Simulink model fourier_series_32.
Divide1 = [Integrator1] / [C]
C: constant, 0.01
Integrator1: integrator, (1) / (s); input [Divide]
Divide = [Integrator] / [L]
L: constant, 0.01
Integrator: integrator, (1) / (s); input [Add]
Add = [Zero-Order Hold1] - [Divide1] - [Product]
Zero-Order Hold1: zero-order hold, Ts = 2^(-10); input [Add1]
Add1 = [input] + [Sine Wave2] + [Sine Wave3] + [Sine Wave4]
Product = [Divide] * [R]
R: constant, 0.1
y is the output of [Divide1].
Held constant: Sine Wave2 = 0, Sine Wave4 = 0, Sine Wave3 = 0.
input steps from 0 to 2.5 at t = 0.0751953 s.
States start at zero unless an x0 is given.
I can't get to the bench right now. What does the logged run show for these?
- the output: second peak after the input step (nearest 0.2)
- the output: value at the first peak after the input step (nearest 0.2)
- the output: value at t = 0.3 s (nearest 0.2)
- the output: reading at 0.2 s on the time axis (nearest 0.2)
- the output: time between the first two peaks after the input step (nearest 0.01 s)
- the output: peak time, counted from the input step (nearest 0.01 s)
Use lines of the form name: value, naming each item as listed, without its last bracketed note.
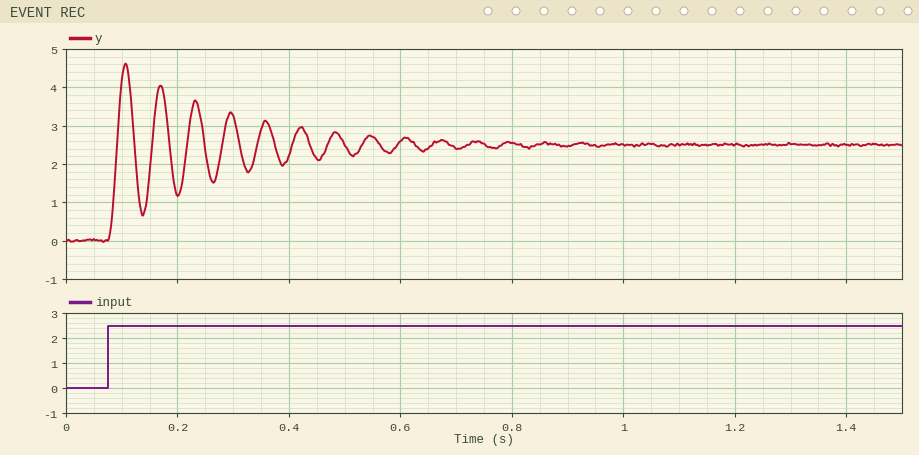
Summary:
the output: second peak after the input step: 4.0
the output: value at the first peak after the input step: 4.6
the output: value at t = 0.3 s: 3.2
the output: reading at 0.2 s on the time axis: 1.2
the output: time between the first two peaks after the input step: 0.06 s
the output: peak time, counted from the input step: 0.03 s
